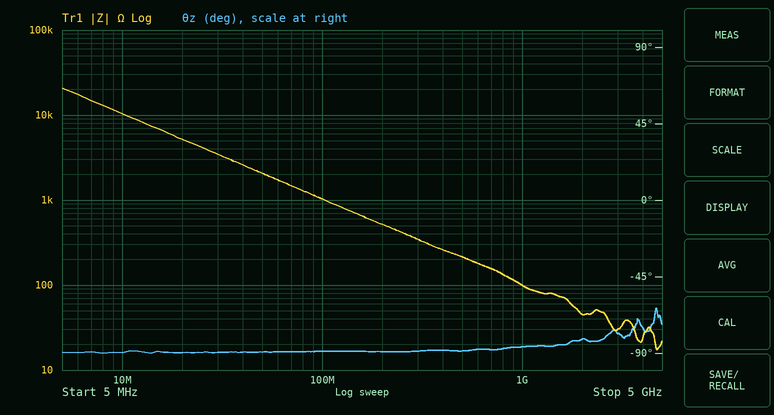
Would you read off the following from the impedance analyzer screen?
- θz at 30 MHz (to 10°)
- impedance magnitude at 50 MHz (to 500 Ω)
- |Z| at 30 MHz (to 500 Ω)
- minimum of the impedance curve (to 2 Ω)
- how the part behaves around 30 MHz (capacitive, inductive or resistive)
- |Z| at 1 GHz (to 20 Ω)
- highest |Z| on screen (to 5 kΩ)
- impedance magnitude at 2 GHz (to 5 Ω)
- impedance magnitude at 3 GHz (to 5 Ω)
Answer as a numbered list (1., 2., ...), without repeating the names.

1. -90°
2. 2.0 kΩ
3. 3.5 kΩ
4. 18 Ω
5. capacitive
6. 100 Ω
7. 20 kΩ
8. 45 Ω
9. 30 Ω
